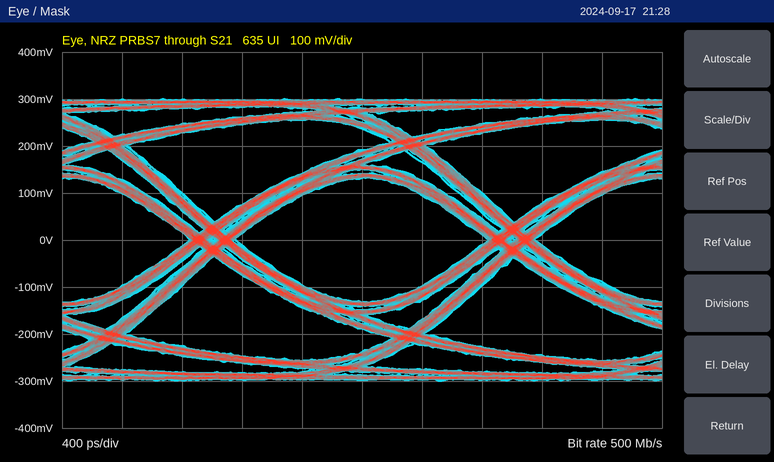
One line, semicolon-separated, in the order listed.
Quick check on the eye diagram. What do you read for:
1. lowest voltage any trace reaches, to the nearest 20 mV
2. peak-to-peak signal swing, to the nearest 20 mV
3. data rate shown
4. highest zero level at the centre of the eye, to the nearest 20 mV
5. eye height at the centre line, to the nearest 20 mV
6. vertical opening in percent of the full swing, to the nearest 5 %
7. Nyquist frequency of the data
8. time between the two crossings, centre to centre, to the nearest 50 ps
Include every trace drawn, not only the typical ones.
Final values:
-300 mV; 600 mV; 500 Mb/s; -140 mV; 260 mV; 45 %; 250 MHz; 2.00 ns
